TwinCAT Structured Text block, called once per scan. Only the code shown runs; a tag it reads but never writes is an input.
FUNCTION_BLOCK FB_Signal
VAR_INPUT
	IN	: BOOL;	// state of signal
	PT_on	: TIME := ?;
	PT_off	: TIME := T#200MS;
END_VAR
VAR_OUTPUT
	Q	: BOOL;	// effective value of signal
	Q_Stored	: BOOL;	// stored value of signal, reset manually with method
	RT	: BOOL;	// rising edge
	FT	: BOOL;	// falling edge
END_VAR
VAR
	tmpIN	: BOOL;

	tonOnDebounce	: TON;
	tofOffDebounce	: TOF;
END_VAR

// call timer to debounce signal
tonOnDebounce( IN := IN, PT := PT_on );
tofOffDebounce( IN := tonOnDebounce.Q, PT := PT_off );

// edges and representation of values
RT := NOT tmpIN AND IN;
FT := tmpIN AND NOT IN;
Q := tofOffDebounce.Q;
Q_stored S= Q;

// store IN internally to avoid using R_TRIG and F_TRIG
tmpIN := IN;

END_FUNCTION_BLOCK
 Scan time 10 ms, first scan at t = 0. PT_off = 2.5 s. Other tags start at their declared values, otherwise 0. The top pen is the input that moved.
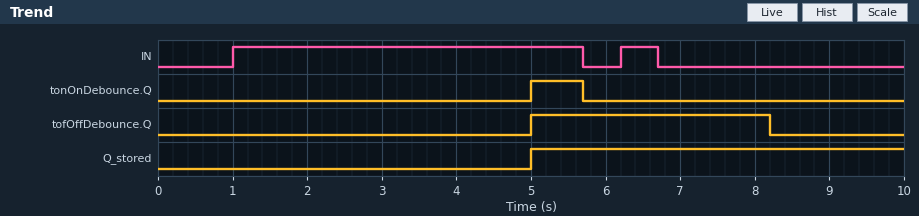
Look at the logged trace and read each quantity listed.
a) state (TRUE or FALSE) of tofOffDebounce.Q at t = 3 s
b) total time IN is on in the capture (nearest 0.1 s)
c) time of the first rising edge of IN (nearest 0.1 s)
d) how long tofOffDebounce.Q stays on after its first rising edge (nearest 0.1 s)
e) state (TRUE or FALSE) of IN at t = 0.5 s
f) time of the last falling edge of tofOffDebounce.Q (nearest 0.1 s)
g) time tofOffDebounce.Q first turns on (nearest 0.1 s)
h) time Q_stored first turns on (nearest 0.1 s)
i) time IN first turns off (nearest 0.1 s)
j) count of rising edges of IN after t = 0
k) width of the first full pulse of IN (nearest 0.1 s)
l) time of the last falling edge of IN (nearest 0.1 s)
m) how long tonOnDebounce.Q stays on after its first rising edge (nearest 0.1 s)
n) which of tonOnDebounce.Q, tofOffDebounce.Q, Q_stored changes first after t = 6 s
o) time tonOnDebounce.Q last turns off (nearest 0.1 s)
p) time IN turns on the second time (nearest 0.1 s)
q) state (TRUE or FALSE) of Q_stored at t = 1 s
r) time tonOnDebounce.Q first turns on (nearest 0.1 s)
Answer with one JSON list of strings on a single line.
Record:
["FALSE", "5.2 s", "1.0 s", "3.2 s", "FALSE", "8.2 s", "5.0 s", "5.0 s", "5.7 s", "2", "4.7 s", "6.7 s", "0.7 s", "tofOffDebounce.Q", "5.7 s", "6.2 s", "FALSE", "5.0 s"]
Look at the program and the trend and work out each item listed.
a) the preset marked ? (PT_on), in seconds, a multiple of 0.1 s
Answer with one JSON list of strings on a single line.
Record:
["4.0 s"]
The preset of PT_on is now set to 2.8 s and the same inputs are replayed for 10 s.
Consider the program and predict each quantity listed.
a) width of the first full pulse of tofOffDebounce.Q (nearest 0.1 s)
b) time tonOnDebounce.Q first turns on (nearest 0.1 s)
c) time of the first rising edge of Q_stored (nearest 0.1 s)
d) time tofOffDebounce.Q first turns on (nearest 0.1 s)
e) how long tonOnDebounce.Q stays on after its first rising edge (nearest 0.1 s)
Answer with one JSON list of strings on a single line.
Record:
["4.4 s", "3.8 s", "3.8 s", "3.8 s", "1.9 s"]
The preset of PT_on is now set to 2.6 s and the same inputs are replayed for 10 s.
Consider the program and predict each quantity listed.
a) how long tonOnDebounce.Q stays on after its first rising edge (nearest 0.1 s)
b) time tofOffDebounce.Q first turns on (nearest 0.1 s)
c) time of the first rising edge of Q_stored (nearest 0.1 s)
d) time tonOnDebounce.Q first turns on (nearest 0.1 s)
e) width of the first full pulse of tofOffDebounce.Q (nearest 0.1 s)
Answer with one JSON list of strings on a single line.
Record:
["2.1 s", "3.6 s", "3.6 s", "3.6 s", "4.6 s"]
